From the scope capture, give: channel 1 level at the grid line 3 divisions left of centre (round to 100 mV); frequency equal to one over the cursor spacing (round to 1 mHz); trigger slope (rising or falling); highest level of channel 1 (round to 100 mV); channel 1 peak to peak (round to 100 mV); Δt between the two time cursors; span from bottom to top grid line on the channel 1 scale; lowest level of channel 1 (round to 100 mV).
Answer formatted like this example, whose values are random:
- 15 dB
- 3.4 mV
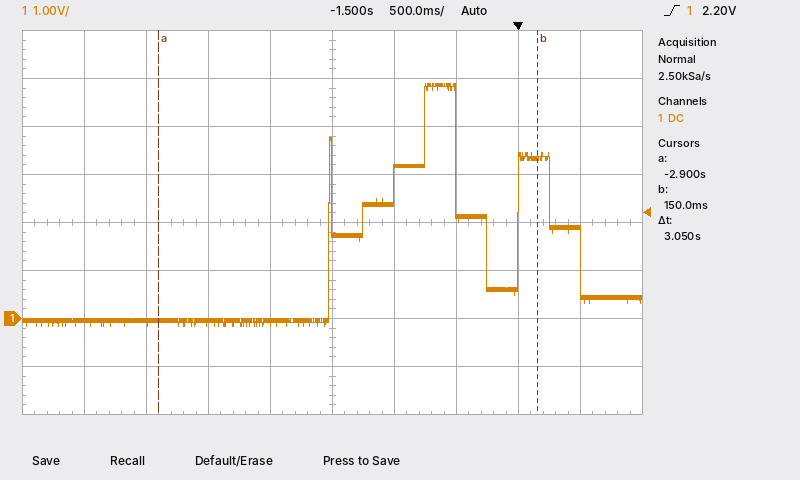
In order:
- -100 mV
- 328 mHz
- rising
- 4.9 V
- 5.1 V
- 3.05 s
- 8 V
- -200 mV
